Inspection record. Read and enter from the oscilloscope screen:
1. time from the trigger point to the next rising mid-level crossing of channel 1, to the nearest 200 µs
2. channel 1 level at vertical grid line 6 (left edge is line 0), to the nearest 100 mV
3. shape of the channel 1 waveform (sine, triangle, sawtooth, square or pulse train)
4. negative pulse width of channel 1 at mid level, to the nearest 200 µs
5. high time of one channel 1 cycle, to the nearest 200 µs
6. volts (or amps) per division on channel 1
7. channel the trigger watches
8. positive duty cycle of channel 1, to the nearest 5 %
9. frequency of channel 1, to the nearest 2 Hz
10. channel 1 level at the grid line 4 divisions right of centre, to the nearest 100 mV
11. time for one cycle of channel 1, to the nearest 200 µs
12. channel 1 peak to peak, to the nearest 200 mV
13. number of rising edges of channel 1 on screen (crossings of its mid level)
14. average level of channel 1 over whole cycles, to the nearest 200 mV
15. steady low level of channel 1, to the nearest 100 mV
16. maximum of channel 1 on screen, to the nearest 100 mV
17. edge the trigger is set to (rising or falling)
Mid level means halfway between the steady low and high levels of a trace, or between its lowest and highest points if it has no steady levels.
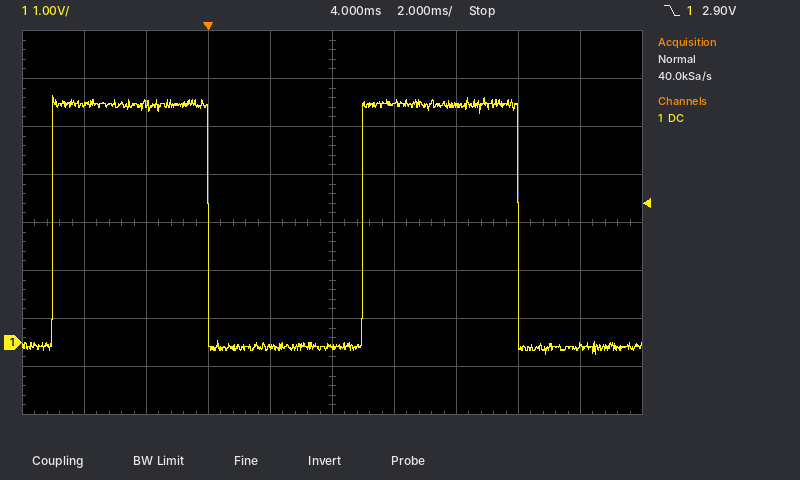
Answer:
5.0 ms
5.0 V
square
5.0 ms
5.0 ms
1 V
channel 1
50 %
100 Hz
-100 mV
10.0 ms
5.4 V
2
2.4 V
-100 mV
5.1 V
falling
